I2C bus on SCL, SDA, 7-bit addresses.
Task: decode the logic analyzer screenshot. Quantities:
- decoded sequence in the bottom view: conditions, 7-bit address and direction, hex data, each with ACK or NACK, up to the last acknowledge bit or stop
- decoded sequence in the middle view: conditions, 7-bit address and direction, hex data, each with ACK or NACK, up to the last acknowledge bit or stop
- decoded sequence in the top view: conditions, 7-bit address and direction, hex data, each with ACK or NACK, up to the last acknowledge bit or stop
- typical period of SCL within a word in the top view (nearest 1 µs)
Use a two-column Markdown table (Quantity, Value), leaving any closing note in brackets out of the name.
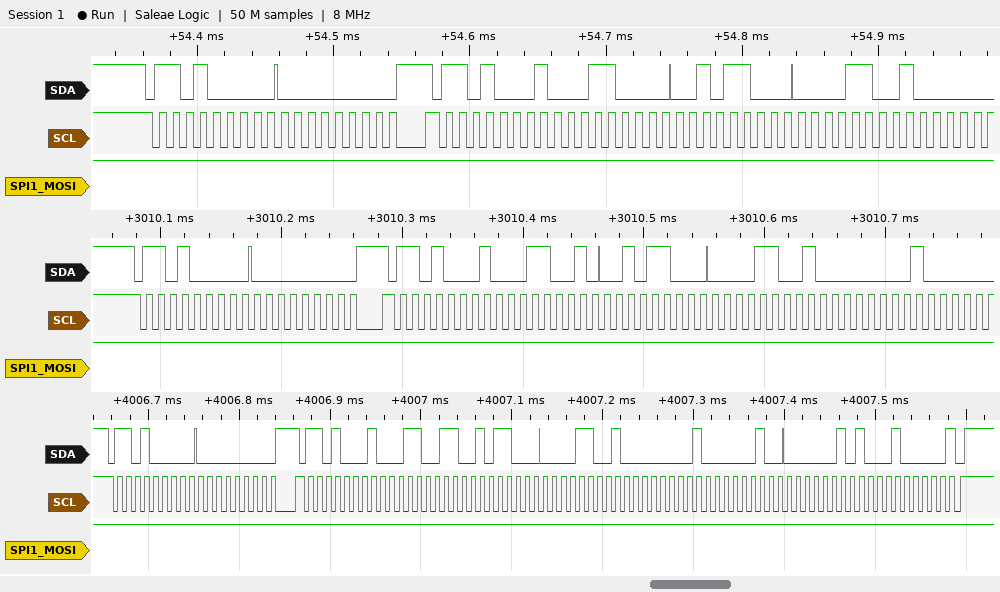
| Quantity | Value |
|---|---|
| decoded sequence in the bottom view: conditions, 7-bit address and direction, hex data, each with ACK or NACK, up to the last acknowledge bit or stop | start, address 68 write ACK, 00 ACK, repeated start, address 68 read ACK, 33 ACK, 58 ACK, 19 ACK, 01 ACK, 04 ACK, 05 ACK, 20 NACK, stop |
| decoded sequence in the middle view: conditions, 7-bit address and direction, hex data, each with ACK or NACK, up to the last acknowledge bit or stop | start, address 68 write ACK, 00 ACK, repeated start, address 68 read ACK, 32 ACK, 58 ACK, 19 ACK, 01 ACK |
| decoded sequence in the top view: conditions, 7-bit address and direction, hex data, each with ACK or NACK, up to the last acknowledge bit or stop | start, address 68 write ACK, 00 ACK, repeated start, address 68 read ACK, 30 ACK, 58 ACK, 19 ACK |
| typical period of SCL within a word in the top view | 10 µs |
